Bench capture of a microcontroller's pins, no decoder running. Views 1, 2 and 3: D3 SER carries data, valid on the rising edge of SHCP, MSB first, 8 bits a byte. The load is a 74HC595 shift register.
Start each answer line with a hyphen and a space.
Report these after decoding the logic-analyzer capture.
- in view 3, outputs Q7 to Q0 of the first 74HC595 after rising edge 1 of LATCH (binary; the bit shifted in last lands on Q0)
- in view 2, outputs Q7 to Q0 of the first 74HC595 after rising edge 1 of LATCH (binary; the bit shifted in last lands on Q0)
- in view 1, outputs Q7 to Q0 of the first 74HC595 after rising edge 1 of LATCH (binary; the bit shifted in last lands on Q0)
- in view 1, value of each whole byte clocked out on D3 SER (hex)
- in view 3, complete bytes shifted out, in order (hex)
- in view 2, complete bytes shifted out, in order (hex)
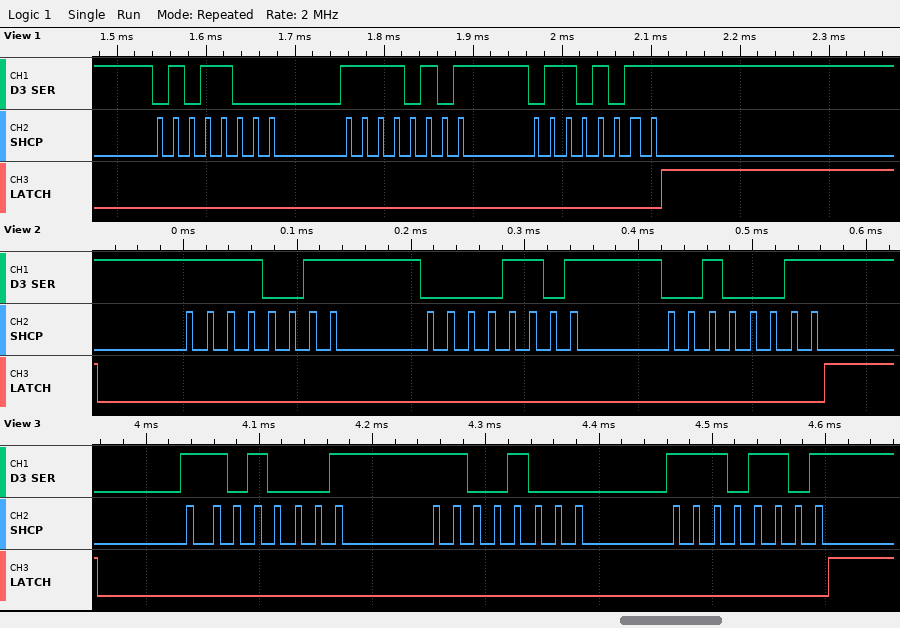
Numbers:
- 11101101
- 00100011
- 01101011
- 58 F5 6B
- D1 C8 ED
- F3 0D 23
